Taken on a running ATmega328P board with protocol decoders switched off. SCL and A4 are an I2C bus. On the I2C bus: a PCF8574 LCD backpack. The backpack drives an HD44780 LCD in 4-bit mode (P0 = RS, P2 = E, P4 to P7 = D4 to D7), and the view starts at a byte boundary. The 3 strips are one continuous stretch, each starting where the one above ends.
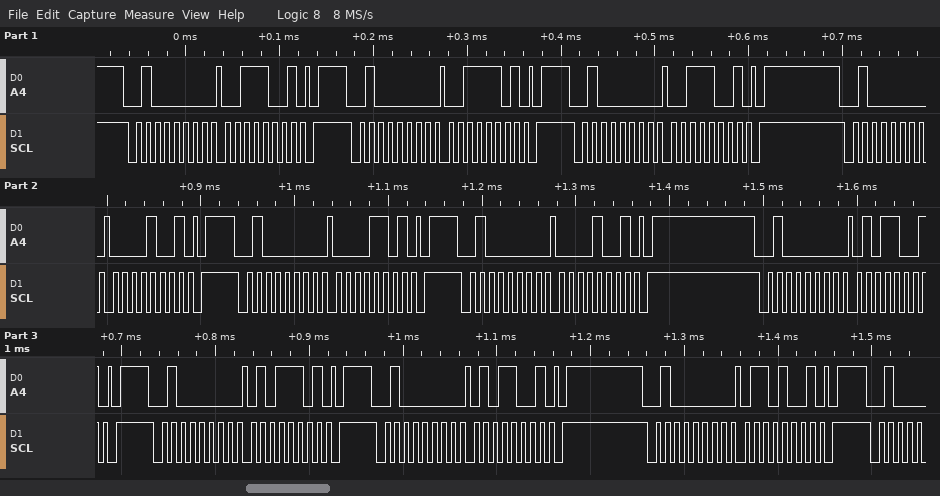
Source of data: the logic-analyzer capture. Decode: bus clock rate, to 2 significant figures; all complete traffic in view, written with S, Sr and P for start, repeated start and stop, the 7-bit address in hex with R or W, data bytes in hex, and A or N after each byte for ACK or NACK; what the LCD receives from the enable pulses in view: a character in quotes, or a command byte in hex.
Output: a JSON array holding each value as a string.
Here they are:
["100 kHz", "S 20W A 39 A P S 20W A 3D A P S 20W A 39 A P S 20W A 09 A P S 20W A 0D A P S 20W A 09 A P S 20W A 59 A P S 20W A 5D A P S 20W A 59 A P S 20W A 69 A P", "'0'"]
